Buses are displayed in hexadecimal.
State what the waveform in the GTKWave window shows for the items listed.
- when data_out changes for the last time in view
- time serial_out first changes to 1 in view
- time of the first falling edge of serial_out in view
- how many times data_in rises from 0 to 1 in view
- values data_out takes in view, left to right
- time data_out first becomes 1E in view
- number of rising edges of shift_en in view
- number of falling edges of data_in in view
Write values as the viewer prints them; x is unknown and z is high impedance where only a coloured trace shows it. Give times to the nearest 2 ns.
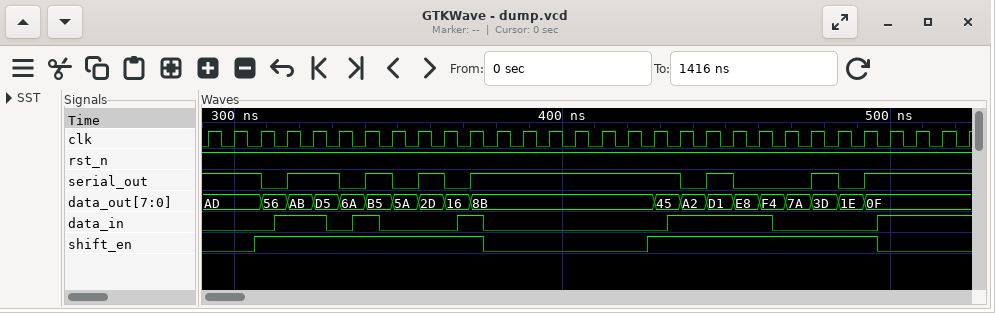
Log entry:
492 ns
316 ns
308 ns
5
AD, 56, AB, D5, 6A, B5, 5A, 2D, 16, 8B, 45, A2, D1, E8, F4, 7A, 3D, 1E, 0F
484 ns
2
4
